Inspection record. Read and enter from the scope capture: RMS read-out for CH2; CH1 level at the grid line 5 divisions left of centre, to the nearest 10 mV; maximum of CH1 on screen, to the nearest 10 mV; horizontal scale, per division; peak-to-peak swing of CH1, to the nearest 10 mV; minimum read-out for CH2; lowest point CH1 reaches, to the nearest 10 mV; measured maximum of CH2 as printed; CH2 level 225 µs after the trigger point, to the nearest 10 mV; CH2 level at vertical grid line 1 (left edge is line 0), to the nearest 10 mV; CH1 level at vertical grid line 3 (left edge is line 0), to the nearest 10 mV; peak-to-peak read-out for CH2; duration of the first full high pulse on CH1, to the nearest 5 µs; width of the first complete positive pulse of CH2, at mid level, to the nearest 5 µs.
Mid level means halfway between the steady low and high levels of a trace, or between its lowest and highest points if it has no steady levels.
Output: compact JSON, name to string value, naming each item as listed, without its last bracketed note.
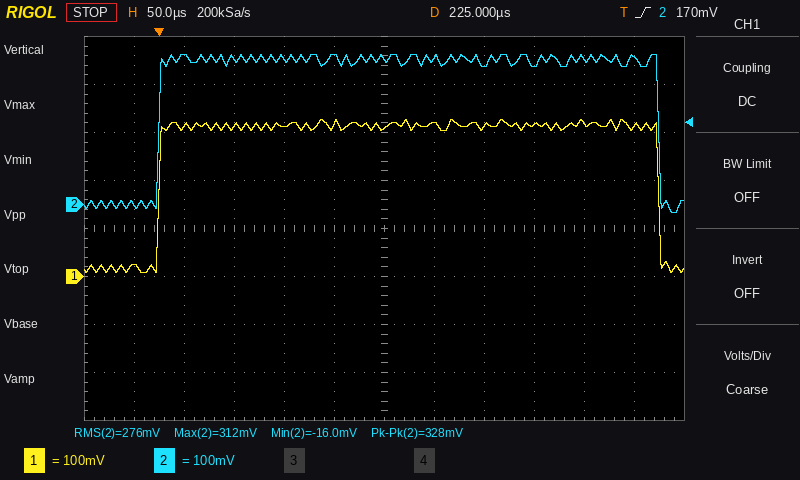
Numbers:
{"RMS read-out for CH2": "276 mV", "CH1 level at the grid line 5 divisions left of centre, to the nearest 10 mV": "20 mV", "maximum of CH1 on screen, to the nearest 10 mV": "330 mV", "horizontal scale, per division": "50 µs", "peak-to-peak swing of CH1, to the nearest 10 mV": "320 mV", "minimum read-out for CH2": "-16.0 mV", "lowest point CH1 reaches, to the nearest 10 mV": "10 mV", "measured maximum of CH2 as printed": "312 mV", "CH2 level 225 µs after the trigger point, to the nearest 10 mV": "300 mV", "CH2 level at vertical grid line 1 (left edge is line 0), to the nearest 10 mV": "0 mV", "CH1 level at vertical grid line 3 (left edge is line 0), to the nearest 10 mV": "310 mV", "peak-to-peak read-out for CH2": "328 mV", "duration of the first full high pulse on CH1, to the nearest 5 µs": "500 µs", "width of the first complete positive pulse of CH2, at mid level, to the nearest 5 µs": "500 µs"}
